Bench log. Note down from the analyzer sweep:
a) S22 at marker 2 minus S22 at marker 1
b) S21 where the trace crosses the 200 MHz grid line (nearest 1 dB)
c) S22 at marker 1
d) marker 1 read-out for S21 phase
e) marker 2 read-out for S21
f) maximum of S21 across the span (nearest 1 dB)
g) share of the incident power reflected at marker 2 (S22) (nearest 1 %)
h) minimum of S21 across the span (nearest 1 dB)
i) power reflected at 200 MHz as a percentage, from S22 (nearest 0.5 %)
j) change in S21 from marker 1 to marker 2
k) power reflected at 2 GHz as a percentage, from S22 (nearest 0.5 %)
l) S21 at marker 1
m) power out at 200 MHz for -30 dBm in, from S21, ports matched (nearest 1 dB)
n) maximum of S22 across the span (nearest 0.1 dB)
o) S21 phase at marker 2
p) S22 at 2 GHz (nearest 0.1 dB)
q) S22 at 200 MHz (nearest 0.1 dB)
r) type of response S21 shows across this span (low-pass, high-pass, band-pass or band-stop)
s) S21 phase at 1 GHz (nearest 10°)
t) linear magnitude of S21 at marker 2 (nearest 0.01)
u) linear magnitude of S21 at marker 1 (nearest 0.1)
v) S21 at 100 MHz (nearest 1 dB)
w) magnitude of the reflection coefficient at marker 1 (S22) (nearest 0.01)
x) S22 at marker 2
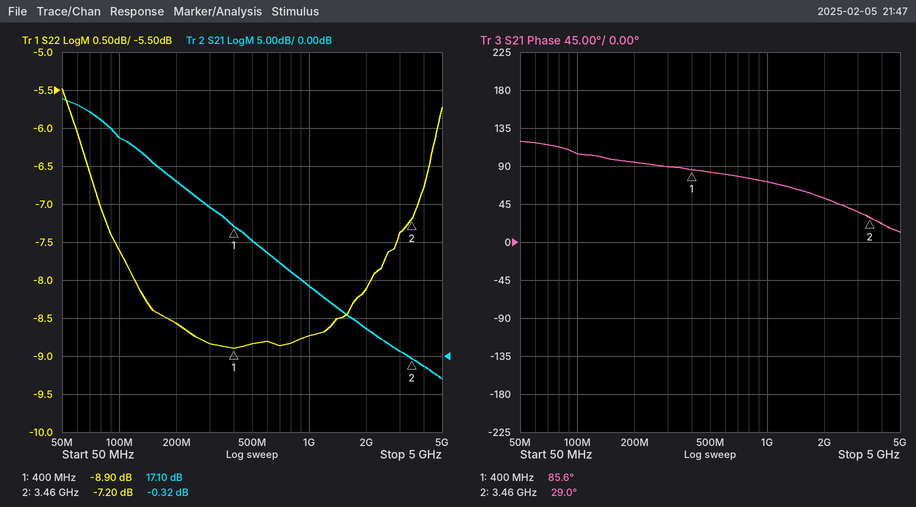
1.70 dB
23 dB
-8.90 dB
85.6°
-0.32 dB
34 dB
19 %
-3 dB
14.0 %
-17.42 dB
15.5 %
17.10 dB
-7 dBm
-5.5 dB
29.0°
-8.1 dB
-8.6 dB
low-pass
70°
0.96
7.2
29 dB
0.36
-7.20 dB
